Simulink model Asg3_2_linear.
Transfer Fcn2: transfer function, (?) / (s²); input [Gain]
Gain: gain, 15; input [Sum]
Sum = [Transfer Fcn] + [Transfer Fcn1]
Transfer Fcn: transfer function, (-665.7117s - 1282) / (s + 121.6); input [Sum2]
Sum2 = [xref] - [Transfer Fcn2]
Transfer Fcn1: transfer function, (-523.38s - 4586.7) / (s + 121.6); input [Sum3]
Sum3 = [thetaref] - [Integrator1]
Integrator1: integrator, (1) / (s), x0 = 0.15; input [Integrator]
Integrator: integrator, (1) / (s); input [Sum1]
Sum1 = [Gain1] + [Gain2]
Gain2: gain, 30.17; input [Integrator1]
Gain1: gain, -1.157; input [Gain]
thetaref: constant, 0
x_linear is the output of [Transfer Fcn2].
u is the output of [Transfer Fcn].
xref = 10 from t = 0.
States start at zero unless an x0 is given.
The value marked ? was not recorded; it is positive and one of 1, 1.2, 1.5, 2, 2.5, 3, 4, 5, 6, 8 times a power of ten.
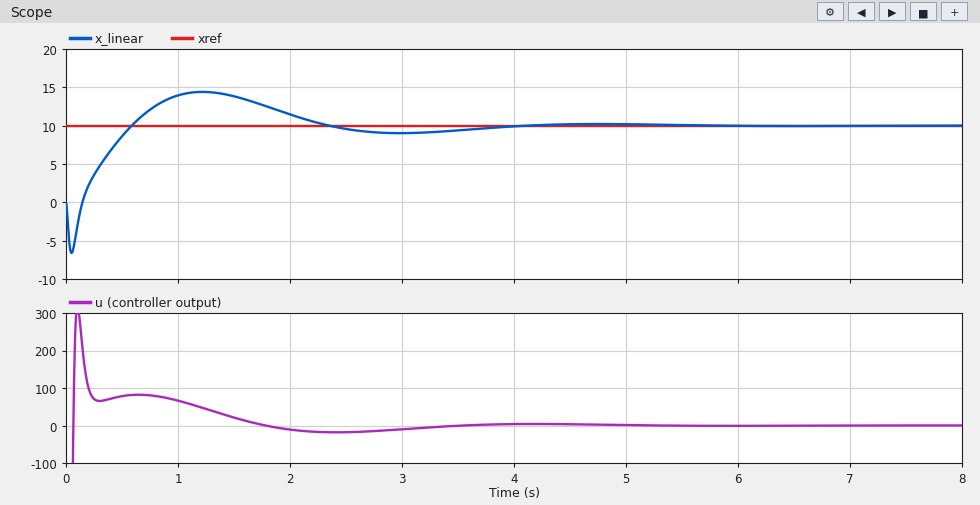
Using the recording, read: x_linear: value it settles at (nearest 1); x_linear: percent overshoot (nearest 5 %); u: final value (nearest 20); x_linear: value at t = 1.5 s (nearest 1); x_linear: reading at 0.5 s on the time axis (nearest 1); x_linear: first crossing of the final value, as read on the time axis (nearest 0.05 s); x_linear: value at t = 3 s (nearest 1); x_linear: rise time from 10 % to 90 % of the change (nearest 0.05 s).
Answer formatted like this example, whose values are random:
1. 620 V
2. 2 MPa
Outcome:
1. 10
2. 45 %
3. 0
4. 14
5. 9
6. 0.60 s
7. 9
8. 0.35 s
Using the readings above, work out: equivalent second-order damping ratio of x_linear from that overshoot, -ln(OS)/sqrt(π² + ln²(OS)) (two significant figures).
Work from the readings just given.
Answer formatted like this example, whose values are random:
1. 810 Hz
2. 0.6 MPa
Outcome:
1. 0.25
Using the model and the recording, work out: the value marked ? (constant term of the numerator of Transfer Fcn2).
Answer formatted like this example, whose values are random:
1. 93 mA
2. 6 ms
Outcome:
1. 0.4
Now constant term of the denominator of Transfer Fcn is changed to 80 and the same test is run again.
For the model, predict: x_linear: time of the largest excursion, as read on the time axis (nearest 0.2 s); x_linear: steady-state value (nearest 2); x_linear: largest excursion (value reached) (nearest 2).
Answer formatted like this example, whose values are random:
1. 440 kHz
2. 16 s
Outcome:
1. 0.8 s
2. 10
3. 14
